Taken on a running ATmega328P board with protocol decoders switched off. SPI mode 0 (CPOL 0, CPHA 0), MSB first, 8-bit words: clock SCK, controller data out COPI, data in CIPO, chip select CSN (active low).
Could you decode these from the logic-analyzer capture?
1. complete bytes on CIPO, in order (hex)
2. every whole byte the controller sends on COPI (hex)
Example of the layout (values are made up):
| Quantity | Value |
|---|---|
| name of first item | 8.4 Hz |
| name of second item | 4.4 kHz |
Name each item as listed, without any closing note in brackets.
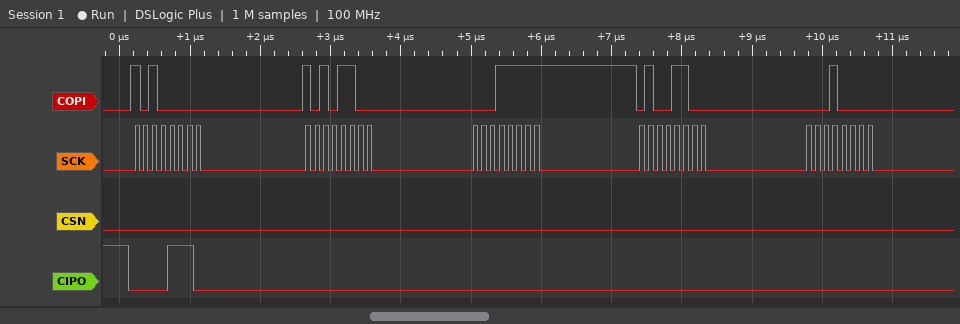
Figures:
| Quantity | Value |
|---|---|
| complete bytes on CIPO, in order | 0E 00 00 00 00 |
| every whole byte the controller sends on COPI | A0 AC 1F 4C 10 |
